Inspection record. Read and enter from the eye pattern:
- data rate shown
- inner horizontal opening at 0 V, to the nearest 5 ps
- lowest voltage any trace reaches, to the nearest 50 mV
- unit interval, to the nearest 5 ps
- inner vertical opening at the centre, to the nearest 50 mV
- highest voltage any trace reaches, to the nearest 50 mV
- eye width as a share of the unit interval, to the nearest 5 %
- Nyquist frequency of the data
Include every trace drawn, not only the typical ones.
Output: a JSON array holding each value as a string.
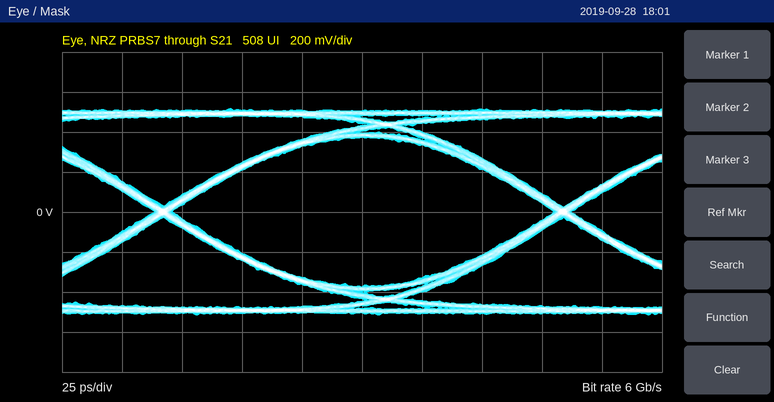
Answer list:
["6 Gb/s", "160 ps", "-500 mV", "165 ps", "750 mV", "500 mV", "95 %", "3 GHz"]
